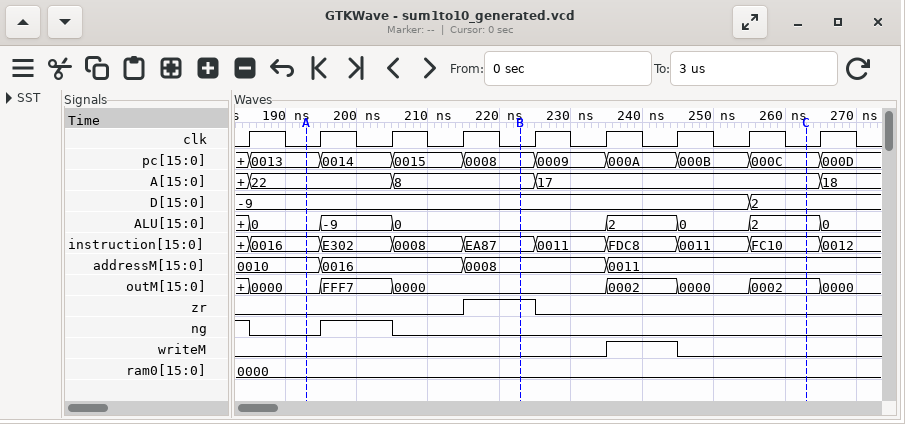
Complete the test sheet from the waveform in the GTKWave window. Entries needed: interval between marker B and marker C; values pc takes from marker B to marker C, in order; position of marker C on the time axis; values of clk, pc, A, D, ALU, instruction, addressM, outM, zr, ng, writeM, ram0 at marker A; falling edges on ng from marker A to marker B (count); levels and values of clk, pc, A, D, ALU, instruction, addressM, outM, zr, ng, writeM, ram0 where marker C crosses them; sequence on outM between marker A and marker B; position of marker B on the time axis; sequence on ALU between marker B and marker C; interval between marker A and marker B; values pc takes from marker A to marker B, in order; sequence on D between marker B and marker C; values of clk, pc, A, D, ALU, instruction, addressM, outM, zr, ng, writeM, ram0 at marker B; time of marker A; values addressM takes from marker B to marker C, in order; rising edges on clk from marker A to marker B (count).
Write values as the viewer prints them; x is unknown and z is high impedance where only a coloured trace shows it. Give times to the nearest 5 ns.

40 ns
0008, 0009, 000A, 000B, 000C
265 ns
clk=0, pc=0013, A=22, D=-9, ALU=0, instruction=0016, addressM=0010, outM=0000, zr=0, ng=0, writeM=0, ram0=0000
1
clk=0, pc=000C, A=17, D=2, ALU=2, instruction=FC10, addressM=0011, outM=0002, zr=0, ng=0, writeM=0, ram0=0000
0000, FFF7, 0000
225 ns
0, 2, 0, 2
30 ns
0013, 0014, 0015, 0008
-9, 2
clk=0, pc=0008, A=8, D=-9, ALU=0, instruction=EA87, addressM=0008, outM=0000, zr=1, ng=0, writeM=0, ram0=0000
195 ns
0008, 0011
3
